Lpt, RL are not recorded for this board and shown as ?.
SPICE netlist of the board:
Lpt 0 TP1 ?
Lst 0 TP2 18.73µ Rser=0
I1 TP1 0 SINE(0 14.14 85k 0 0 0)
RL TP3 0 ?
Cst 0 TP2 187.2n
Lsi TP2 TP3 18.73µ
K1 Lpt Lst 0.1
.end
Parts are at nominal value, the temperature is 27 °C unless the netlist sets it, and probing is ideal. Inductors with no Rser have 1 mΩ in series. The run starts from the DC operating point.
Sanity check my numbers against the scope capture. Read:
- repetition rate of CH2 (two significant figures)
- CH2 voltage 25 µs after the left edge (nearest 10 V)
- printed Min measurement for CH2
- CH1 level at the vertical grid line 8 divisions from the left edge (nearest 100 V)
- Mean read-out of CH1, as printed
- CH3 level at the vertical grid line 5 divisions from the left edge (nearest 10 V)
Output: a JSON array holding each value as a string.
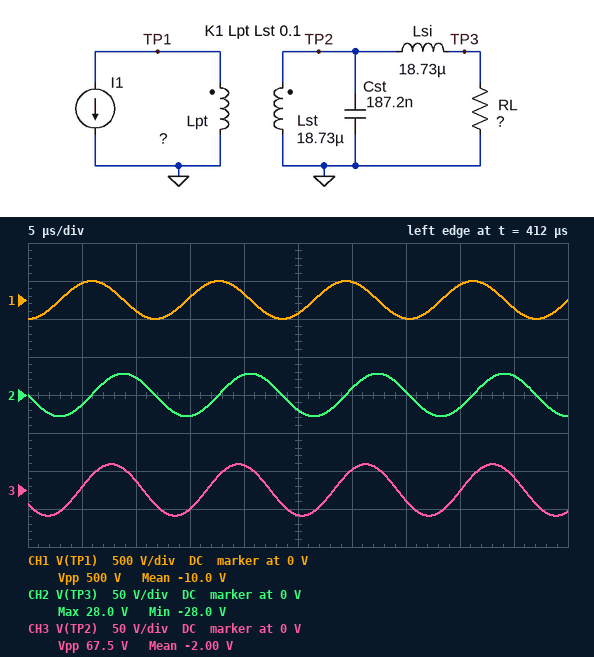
["85 kHz", "-20 V", "-28.0 V", "200 V", "-10.0 V", "-30 V"]
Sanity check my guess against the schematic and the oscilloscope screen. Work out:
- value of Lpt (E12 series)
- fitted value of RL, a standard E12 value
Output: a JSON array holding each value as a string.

["33 µH", "15 Ω"]
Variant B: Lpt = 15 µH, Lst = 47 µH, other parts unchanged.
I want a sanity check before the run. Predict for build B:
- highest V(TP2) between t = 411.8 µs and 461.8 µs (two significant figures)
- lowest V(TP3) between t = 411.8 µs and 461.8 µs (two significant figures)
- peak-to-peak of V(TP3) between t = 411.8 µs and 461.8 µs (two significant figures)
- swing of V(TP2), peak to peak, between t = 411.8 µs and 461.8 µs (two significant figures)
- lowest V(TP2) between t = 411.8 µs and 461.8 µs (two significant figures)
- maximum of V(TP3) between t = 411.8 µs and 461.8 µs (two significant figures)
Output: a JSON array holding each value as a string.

["15 V", "-12 V", "24 V", "29 V", "-15 V", "12 V"]
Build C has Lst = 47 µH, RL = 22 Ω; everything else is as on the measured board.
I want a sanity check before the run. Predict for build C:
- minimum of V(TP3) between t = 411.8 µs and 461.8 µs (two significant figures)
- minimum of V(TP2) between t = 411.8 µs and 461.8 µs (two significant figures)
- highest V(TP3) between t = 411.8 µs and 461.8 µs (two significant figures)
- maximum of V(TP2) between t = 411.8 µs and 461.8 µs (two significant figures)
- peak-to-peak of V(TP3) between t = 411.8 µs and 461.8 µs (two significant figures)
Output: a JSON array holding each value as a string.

["-19 V", "-21 V", "19 V", "21 V", "38 V"]
